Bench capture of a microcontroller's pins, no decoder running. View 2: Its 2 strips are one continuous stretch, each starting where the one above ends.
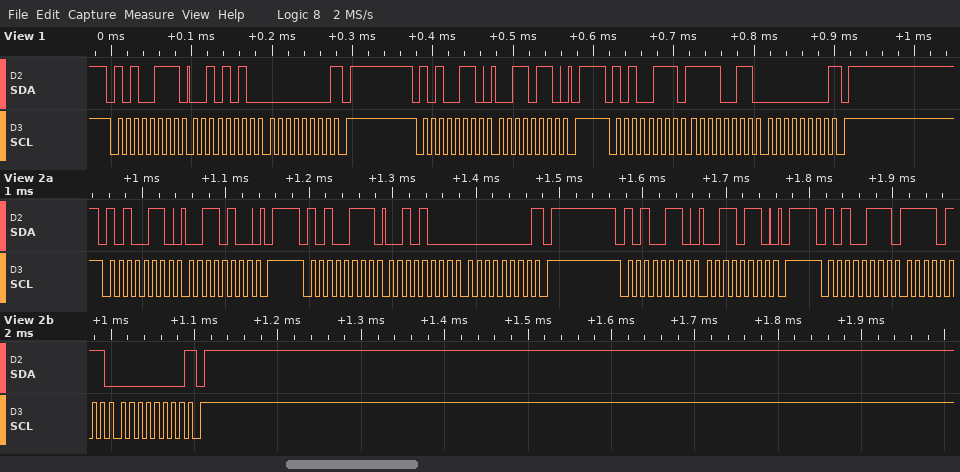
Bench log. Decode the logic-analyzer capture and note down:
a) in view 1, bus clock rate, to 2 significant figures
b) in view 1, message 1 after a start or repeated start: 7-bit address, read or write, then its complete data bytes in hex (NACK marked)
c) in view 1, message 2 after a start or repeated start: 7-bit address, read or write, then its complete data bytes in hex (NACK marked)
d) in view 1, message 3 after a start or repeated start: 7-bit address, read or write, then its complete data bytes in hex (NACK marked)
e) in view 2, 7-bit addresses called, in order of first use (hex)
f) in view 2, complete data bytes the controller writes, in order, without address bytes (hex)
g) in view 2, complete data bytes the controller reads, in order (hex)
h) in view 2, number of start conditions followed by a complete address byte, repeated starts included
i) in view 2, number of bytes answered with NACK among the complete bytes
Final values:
100 kHz
0x53 read: 2A 00 NACK
0x53 write: 36
0x53 read: F3 00 NACK
0x53
34 36
28 00 F7 00
4
2
